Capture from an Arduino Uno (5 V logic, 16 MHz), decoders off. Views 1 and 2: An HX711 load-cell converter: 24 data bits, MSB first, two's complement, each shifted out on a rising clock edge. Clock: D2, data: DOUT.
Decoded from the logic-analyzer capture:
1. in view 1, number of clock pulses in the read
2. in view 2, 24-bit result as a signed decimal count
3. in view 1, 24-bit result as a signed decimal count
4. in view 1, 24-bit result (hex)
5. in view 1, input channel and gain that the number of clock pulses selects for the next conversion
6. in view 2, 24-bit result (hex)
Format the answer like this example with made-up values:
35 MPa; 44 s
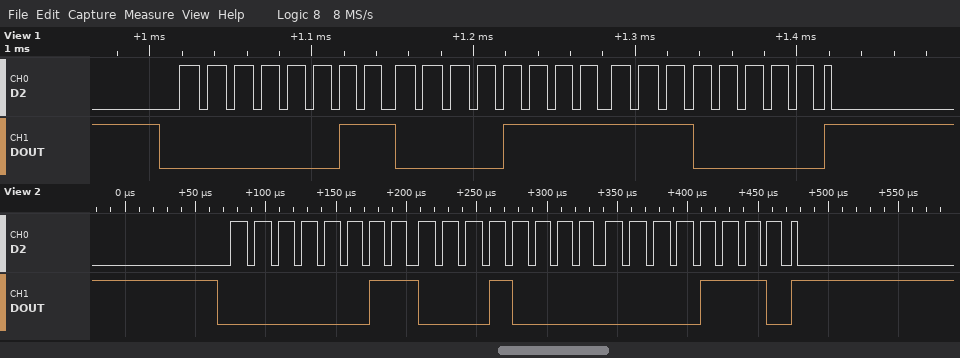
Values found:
25; 200718; 200672; 0x030FE0; channel A, gain 128; 0x03100E
